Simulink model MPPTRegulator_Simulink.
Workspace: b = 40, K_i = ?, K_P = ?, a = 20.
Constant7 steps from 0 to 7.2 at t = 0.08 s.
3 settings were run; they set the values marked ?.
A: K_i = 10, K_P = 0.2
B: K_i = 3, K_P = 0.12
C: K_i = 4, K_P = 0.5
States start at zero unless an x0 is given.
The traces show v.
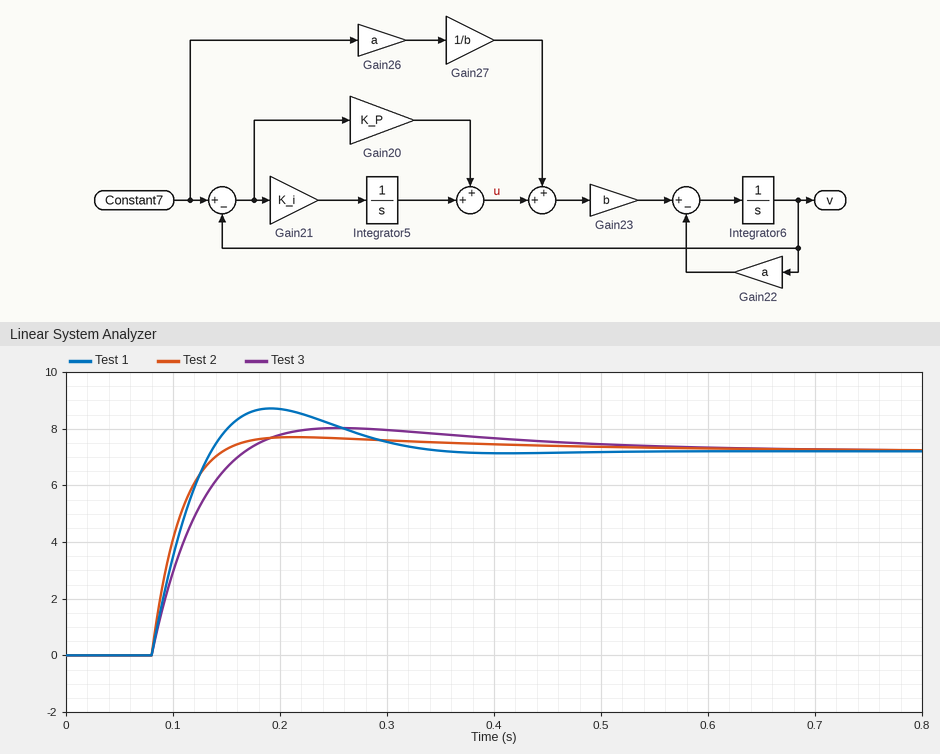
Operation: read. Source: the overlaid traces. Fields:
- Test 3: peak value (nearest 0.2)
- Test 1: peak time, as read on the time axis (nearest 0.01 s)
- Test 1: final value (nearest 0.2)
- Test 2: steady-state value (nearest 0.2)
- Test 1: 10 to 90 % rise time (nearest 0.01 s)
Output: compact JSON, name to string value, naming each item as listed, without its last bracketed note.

{"Test 3: peak value": "8.0", "Test 1: peak time, as read on the time axis": "0.19 s", "Test 1: final value": "7.2", "Test 2: steady-state value": "7.2", "Test 1: 10 to 90 % rise time": "0.04 s"}
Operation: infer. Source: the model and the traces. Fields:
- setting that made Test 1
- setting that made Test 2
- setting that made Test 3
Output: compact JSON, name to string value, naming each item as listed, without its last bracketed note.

{"setting that made Test 1": "A", "setting that made Test 2": "C", "setting that made Test 3": "B"}
